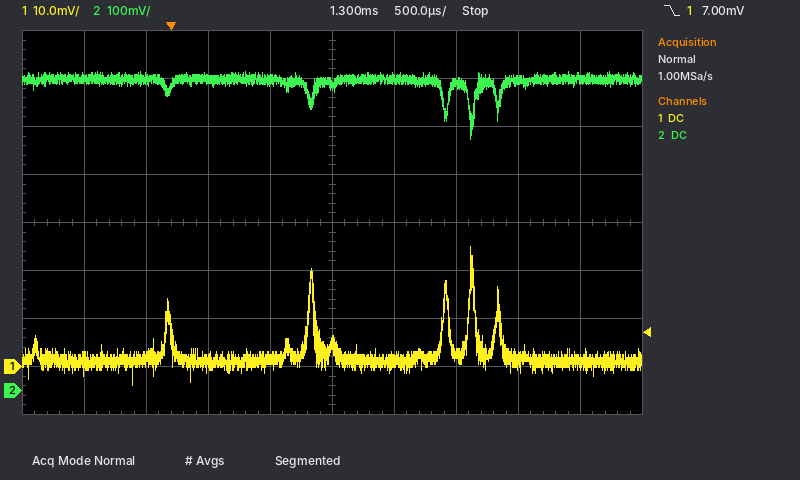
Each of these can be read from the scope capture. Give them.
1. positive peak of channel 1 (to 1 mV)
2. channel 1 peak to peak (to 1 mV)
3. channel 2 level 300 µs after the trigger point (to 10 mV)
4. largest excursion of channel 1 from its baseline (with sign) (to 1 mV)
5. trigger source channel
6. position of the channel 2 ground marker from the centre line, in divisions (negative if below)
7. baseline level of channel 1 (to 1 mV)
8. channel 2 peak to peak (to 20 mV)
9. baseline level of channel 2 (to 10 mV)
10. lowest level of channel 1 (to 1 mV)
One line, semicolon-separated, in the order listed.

25 mV; 29 mV; 650 mV; +24 mV; channel 1; -3.5 div; 1 mV; 140 mV; 650 mV; -4 mV
